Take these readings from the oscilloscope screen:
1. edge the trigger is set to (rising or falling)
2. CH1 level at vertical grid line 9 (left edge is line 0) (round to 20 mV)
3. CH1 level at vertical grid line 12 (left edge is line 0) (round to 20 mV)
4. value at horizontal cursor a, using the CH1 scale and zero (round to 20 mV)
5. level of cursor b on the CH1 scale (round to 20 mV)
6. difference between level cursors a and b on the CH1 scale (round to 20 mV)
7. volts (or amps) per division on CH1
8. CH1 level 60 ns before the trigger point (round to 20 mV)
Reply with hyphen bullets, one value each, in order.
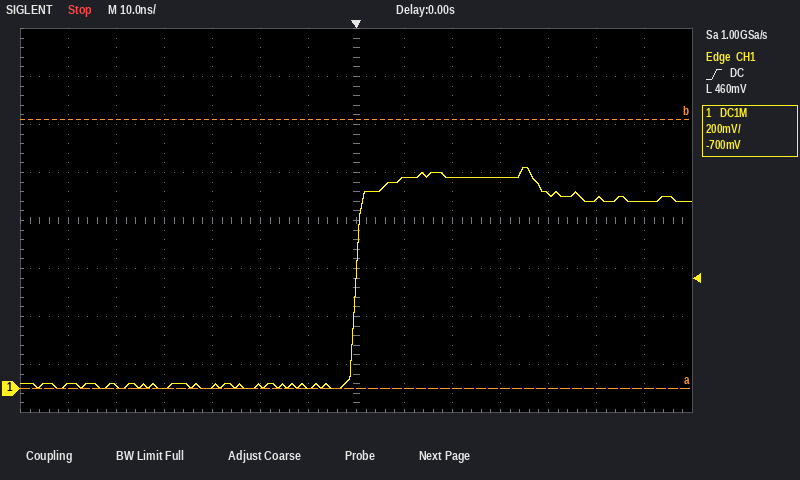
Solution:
- rising
- 880 mV
- 780 mV
- 0 mV
- 1.12 V
- 1.12 V
- 200 mV
- 20 mV
